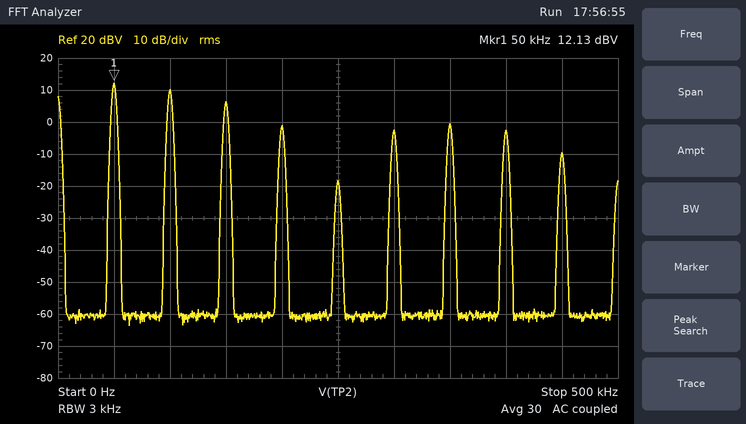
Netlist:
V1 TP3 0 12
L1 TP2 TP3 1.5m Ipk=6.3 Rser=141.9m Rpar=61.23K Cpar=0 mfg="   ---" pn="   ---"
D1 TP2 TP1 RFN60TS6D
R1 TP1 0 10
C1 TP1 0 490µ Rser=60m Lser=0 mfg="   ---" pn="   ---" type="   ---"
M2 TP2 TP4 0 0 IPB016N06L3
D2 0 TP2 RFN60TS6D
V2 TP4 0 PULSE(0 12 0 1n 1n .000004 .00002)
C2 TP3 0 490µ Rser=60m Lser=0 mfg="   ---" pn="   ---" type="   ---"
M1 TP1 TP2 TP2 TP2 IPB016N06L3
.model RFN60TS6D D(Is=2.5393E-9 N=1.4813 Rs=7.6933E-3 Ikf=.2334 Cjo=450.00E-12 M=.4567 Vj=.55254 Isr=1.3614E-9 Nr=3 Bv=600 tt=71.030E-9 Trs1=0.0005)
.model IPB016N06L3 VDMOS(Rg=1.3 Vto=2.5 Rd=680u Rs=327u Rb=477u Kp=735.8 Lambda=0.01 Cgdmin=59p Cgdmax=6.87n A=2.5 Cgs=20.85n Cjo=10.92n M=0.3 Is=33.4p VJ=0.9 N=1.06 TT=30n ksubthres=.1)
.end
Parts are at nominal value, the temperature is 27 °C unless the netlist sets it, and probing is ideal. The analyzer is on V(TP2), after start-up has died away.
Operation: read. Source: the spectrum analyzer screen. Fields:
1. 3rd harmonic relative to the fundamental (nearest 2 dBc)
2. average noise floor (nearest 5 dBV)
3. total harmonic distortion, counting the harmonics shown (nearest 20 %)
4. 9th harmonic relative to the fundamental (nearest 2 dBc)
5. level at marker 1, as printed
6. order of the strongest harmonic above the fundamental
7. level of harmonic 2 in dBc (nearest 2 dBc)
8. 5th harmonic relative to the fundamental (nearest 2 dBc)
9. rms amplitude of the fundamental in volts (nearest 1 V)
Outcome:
-6 dBc
-60 dBV
100 %
-22 dBc
12.13 dBV
2
-2 dBc
-30 dBc
4 V
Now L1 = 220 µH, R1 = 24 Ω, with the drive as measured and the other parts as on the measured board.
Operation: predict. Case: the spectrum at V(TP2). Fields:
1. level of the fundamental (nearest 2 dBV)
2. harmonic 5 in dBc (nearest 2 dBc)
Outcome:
12 dBV
-26 dBc
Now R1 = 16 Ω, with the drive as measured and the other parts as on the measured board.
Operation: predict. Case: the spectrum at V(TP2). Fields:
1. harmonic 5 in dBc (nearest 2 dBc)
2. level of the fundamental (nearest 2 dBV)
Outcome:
-28 dBc
12 dBV
